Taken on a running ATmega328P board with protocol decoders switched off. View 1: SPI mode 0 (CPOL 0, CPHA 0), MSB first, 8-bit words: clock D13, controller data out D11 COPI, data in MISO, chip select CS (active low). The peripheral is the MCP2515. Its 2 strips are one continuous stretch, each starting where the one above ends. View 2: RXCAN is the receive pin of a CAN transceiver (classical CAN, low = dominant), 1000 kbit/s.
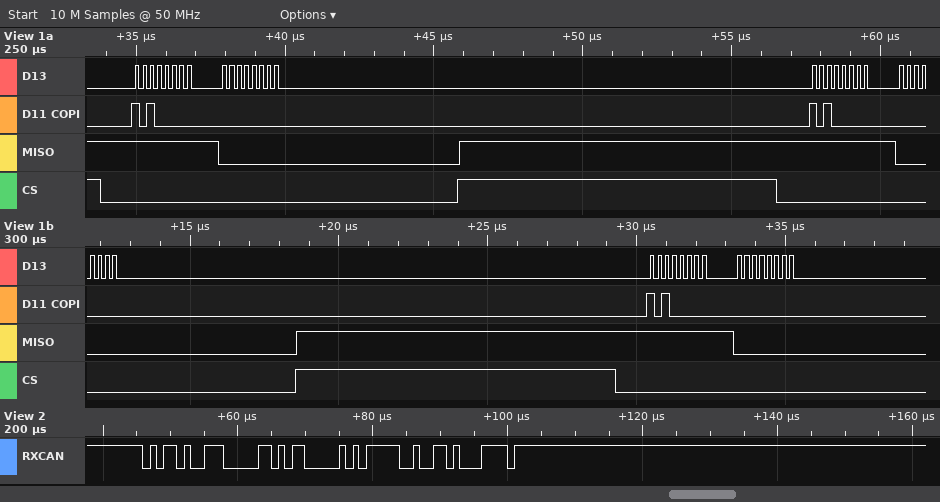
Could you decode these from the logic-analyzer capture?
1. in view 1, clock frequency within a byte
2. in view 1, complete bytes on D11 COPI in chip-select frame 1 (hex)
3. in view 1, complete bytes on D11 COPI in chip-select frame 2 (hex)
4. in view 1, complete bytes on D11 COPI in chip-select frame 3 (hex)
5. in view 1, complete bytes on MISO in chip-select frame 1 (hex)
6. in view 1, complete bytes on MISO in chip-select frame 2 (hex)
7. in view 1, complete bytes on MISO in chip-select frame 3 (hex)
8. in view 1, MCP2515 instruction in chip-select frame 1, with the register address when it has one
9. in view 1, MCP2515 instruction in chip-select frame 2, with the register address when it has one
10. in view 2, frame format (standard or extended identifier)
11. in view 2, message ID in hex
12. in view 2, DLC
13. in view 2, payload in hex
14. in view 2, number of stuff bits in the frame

4 MHz
0xA0 0x00
0xA0 0x00
0xA0 0x00
0xFF 0x00
0xFF 0x00
0xFF 0x00
READ STATUS
READ STATUS
standard
0x5A7
2
B0 2F
3
